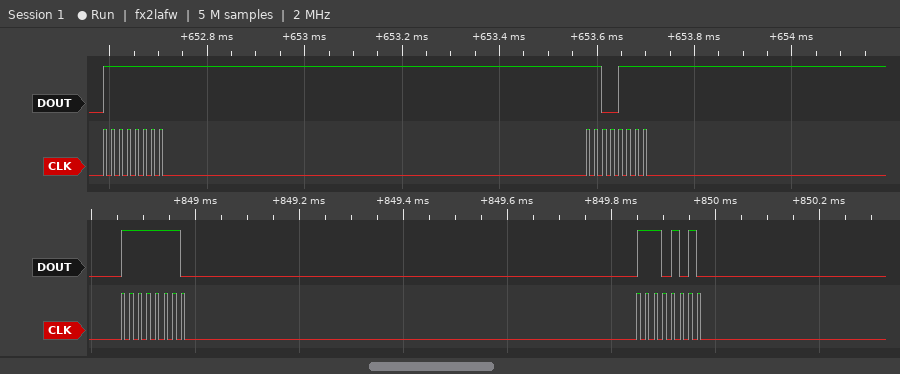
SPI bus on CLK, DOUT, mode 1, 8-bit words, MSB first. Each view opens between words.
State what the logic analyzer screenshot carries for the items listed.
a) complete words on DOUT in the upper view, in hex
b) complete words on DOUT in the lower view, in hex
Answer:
FF, CF
FE, EA
